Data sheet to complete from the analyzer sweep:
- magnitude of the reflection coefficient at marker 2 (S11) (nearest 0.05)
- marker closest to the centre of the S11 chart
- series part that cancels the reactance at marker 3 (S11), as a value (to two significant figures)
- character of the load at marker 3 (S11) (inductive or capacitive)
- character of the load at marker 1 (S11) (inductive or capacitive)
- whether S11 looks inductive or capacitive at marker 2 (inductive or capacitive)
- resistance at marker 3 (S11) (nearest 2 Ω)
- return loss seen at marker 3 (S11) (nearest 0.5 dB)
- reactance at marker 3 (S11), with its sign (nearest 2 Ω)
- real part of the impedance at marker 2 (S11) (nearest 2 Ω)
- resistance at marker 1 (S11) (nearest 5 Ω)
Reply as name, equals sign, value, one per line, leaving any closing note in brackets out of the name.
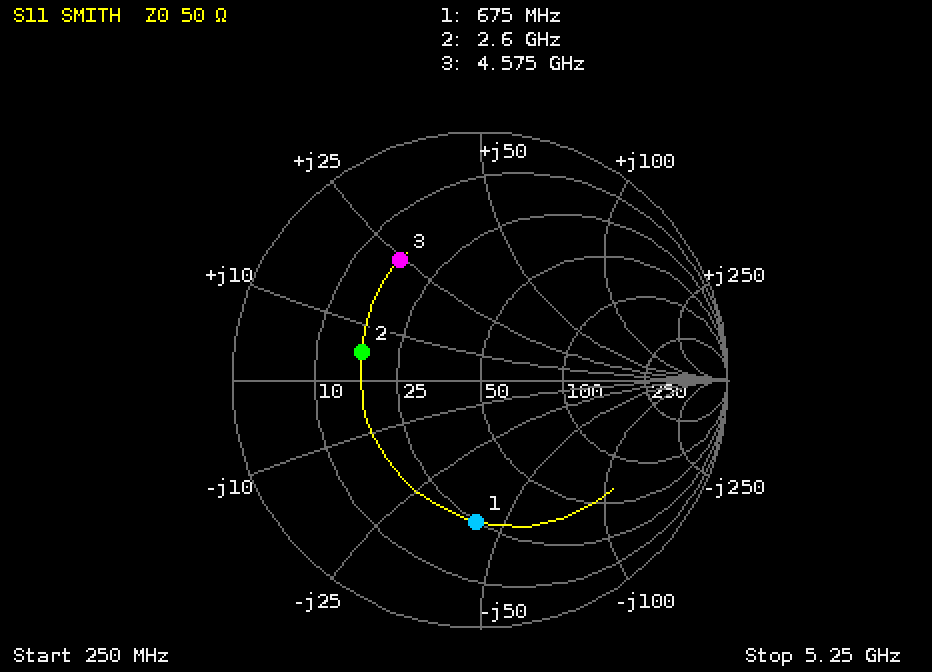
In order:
magnitude of the reflection coefficient at marker 2 (S11) = 0.50
marker closest to the centre of the S11 chart = marker 2
series part that cancels the reactance at marker 3 (S11), as a value = 1.4 pF
character of the load at marker 3 (S11) = inductive
character of the load at marker 1 (S11) = capacitive
whether S11 looks inductive or capacitive at marker 2 = inductive
resistance at marker 3 (S11) = 16 Ω
return loss seen at marker 3 (S11) = 4.5 dB
reactance at marker 3 (S11), with its sign = +24 Ω
real part of the impedance at marker 2 (S11) = 18 Ω
resistance at marker 1 (S11) = 25 Ω
